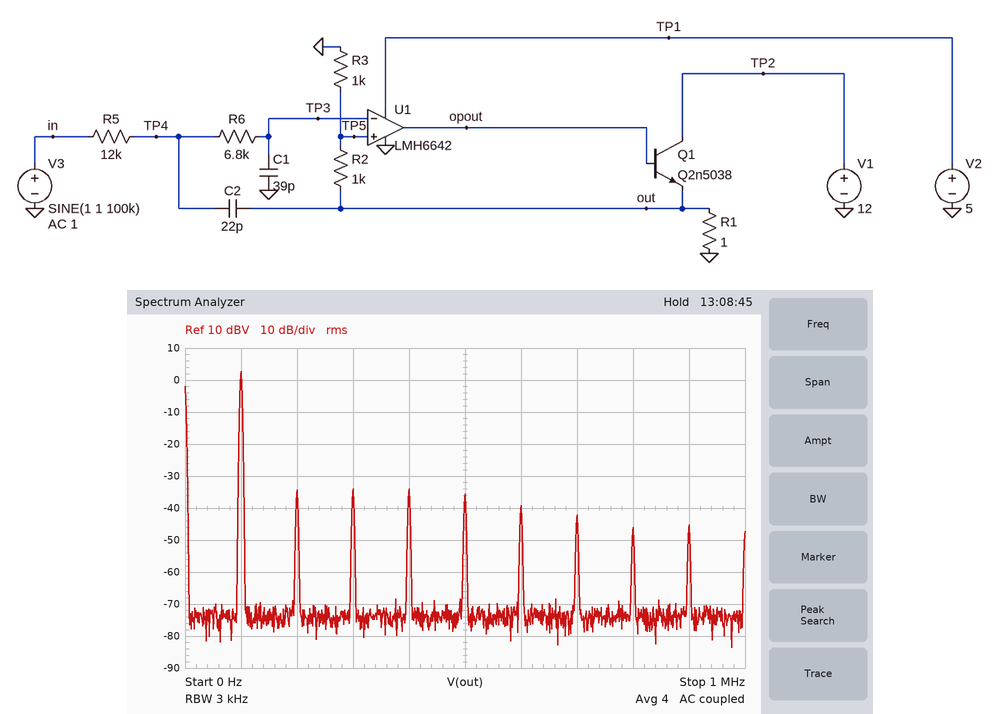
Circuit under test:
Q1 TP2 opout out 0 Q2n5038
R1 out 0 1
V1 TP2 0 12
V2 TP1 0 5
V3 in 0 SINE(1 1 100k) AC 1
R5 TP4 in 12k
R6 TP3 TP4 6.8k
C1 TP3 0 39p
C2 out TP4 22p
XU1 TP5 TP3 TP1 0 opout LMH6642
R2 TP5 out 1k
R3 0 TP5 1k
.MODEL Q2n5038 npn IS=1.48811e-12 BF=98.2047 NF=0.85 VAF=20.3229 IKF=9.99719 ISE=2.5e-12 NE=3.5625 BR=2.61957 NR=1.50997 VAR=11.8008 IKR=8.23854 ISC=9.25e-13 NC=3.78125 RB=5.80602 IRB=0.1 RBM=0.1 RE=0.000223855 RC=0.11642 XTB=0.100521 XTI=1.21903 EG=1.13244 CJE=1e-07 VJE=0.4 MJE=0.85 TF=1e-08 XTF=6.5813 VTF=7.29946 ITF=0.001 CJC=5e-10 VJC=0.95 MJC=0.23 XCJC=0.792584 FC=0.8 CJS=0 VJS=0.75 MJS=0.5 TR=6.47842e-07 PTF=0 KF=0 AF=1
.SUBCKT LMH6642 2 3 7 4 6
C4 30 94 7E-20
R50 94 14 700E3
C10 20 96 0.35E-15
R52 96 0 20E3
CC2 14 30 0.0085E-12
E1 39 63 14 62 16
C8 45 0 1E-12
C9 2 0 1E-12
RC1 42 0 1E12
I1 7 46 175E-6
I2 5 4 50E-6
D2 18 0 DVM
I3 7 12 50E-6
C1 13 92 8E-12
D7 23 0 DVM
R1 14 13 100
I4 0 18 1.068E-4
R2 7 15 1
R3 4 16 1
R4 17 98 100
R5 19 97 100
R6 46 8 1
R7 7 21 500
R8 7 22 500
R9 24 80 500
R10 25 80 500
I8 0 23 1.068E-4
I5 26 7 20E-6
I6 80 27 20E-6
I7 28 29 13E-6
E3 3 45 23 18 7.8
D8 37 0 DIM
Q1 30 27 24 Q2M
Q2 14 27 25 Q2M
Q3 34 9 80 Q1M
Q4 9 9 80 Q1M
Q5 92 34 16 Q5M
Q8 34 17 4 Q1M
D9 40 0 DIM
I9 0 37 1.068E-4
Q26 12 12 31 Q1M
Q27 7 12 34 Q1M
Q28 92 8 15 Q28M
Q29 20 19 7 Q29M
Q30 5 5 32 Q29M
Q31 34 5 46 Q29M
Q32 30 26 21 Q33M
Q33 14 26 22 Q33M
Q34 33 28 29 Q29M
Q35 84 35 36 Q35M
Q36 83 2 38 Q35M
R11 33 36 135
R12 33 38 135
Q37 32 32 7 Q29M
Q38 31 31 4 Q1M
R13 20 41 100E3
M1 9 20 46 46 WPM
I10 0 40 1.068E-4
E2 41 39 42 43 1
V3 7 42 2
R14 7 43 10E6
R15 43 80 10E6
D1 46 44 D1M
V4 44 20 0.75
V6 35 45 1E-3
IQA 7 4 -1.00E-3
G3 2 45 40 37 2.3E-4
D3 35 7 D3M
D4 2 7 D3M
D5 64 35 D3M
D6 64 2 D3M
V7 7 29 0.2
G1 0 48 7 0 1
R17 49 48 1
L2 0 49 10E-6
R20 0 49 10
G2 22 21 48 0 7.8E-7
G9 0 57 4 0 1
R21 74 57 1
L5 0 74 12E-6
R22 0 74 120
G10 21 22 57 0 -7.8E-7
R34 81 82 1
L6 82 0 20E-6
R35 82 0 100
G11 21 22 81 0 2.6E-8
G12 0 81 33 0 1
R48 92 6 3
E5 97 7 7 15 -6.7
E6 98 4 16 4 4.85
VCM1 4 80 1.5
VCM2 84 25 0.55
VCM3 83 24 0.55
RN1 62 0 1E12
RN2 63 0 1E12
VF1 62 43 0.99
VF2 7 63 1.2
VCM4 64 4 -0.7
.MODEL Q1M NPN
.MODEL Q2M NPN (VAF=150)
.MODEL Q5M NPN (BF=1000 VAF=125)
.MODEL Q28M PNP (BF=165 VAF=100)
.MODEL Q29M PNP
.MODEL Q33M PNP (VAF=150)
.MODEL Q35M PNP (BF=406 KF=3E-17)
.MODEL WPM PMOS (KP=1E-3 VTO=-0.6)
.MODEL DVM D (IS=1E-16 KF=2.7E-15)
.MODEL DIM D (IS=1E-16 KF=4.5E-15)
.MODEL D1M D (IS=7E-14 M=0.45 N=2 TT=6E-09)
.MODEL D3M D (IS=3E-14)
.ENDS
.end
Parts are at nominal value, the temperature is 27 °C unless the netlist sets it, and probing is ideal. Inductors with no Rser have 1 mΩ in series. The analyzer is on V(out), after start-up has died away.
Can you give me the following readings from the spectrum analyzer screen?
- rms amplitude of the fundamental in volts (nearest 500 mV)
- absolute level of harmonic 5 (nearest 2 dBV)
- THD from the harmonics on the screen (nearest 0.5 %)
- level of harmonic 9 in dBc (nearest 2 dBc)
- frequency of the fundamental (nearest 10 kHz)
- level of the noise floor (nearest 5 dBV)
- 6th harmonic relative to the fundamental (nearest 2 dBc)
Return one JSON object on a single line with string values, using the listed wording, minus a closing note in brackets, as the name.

{"rms amplitude of the fundamental in volts": "1.5 V", "absolute level of harmonic 5": "-36 dBV", "THD from the harmonics on the screen": "3.0 %", "level of harmonic 9 in dBc": "-48 dBc", "frequency of the fundamental": "100 kHz", "level of the noise floor": "-75 dBV", "6th harmonic relative to the fundamental": "-42 dBc"}
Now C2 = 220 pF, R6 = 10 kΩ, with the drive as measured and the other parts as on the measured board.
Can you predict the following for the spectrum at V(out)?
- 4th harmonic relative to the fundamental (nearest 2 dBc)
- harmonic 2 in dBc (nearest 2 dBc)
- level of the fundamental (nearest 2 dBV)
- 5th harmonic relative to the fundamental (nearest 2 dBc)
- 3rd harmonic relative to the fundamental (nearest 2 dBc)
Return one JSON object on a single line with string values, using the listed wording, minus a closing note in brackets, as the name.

{"4th harmonic relative to the fundamental": "-24 dBc", "harmonic 2 in dBc": "-16 dBc", "level of the fundamental": "4 dBV", "5th harmonic relative to the fundamental": "-30 dBc", "3rd harmonic relative to the fundamental": "-18 dBc"}
